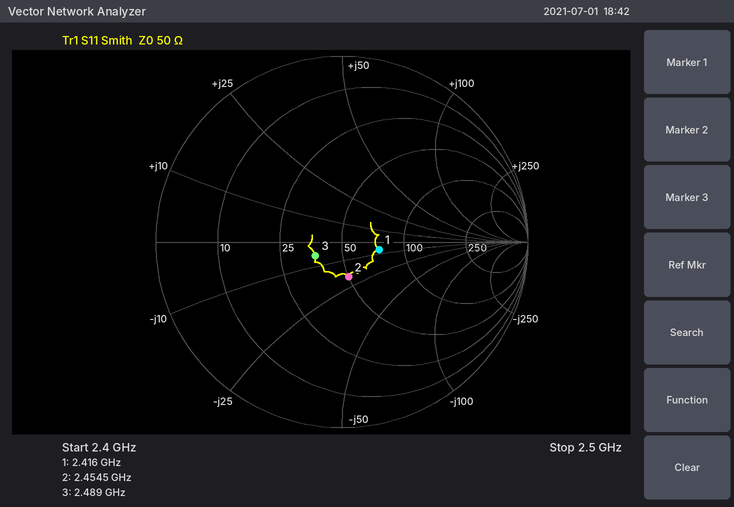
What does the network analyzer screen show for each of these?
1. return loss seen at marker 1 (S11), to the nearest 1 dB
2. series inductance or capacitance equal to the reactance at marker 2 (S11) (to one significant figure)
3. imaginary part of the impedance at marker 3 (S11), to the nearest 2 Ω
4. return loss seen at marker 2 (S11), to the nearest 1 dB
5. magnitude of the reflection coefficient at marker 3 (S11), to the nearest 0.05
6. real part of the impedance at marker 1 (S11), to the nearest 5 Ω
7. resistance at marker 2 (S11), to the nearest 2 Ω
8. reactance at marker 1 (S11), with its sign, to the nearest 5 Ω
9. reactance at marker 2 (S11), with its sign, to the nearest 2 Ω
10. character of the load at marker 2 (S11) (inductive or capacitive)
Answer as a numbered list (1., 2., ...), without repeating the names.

1. 14 dB
2. 3 pF
3. -6 Ω
4. 14 dB
5. 0.15
6. 75 Ω
7. 50 Ω
8. -5 Ω
9. -20 Ω
10. capacitive
